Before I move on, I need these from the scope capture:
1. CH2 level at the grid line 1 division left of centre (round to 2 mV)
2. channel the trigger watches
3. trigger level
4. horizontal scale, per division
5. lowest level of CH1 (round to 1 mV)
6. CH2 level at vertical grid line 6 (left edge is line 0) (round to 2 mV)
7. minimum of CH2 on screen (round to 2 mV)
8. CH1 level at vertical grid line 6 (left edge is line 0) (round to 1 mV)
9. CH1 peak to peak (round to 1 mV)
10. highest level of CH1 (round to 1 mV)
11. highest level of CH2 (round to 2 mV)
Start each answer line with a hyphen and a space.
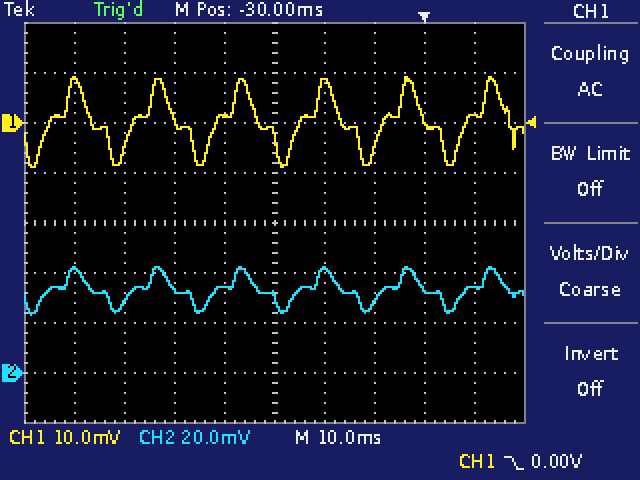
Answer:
- 34 mV
- CH1
- 0.00 V
- 10 ms
- -9 mV
- 42 mV
- 24 mV
- 8 mV
- 18 mV
- 9 mV
- 42 mV
